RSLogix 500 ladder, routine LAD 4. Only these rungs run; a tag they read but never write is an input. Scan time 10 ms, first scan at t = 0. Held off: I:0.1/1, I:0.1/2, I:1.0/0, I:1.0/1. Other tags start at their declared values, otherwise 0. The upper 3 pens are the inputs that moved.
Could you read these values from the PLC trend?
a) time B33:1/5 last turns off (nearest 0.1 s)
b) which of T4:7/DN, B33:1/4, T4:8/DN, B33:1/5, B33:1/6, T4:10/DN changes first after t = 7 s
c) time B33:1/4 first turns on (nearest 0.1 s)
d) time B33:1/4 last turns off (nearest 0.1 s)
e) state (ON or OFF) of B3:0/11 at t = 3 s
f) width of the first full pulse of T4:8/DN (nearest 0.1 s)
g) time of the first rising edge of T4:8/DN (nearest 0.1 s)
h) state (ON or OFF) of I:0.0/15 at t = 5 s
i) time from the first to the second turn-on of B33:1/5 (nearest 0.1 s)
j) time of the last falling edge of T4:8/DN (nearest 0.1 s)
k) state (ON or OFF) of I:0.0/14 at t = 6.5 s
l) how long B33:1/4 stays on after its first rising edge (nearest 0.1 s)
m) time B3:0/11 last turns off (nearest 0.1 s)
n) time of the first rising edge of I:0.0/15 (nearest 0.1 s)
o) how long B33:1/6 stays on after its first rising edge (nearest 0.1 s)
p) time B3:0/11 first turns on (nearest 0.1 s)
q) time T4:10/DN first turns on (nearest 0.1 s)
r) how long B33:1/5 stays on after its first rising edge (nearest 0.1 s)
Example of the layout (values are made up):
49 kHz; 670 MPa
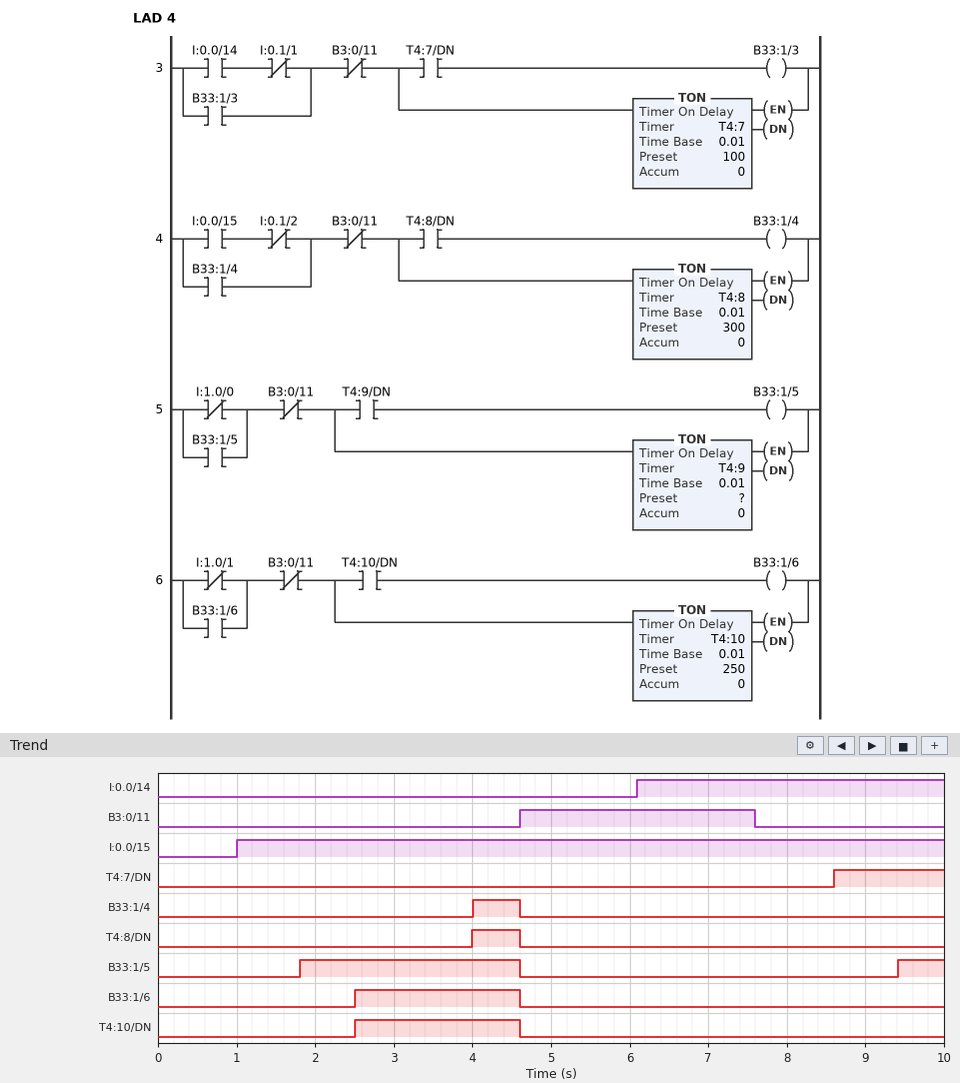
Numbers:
4.6 s; T4:7/DN; 4.0 s; 4.6 s; OFF; 0.6 s; 4.0 s; ON; 7.6 s; 4.6 s; ON; 0.6 s; 7.6 s; 1.0 s; 2.1 s; 4.6 s; 2.5 s; 2.8 s
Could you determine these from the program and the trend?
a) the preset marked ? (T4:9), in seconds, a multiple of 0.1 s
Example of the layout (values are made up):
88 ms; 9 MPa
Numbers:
1.8 s
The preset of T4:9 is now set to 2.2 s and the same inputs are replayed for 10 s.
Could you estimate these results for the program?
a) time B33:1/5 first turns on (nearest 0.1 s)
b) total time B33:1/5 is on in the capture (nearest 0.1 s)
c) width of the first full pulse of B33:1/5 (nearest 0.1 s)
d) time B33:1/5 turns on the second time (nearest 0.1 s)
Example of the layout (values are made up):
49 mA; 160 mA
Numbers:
2.2 s; 2.6 s; 2.4 s; 9.8 s
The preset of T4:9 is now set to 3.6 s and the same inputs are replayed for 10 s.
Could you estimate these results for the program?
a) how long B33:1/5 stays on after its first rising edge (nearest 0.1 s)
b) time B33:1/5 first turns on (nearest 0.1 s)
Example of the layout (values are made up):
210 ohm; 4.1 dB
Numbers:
1.0 s; 3.6 s
